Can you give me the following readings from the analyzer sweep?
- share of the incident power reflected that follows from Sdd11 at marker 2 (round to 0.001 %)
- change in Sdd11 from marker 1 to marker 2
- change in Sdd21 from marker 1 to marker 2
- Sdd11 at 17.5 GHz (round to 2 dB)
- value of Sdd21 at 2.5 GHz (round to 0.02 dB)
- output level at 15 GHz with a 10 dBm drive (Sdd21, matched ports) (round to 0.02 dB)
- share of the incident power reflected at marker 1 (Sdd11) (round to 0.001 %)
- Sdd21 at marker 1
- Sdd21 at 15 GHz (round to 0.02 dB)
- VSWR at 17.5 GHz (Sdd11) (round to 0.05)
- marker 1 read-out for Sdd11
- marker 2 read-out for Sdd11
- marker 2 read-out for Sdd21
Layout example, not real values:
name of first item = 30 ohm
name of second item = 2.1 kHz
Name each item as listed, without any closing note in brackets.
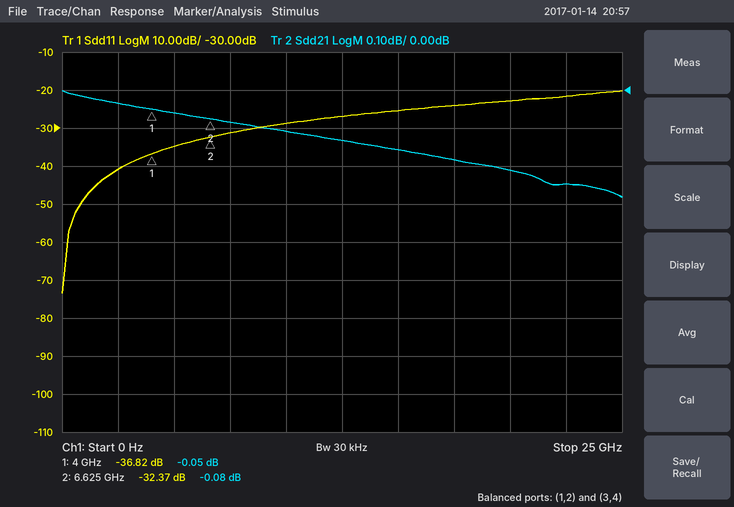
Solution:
share of the incident power reflected that follows from Sdd11 at marker 2 = 0.058 %
change in Sdd11 from marker 1 to marker 2 = 4.45 dB
change in Sdd21 from marker 1 to marker 2 = -0.03 dB
Sdd11 at 17.5 GHz = -24 dB
value of Sdd21 at 2.5 GHz = -0.04 dB
output level at 15 GHz with a 10 dBm drive (Sdd21, matched ports) = 9.84 dBm
share of the incident power reflected at marker 1 (Sdd11) = 0.021 %
Sdd21 at marker 1 = -0.05 dB
Sdd21 at 15 GHz = -0.16 dB
VSWR at 17.5 GHz (Sdd11) = 1.15
marker 1 read-out for Sdd11 = -36.82 dB
marker 2 read-out for Sdd11 = -32.37 dB
marker 2 read-out for Sdd21 = -0.08 dB
